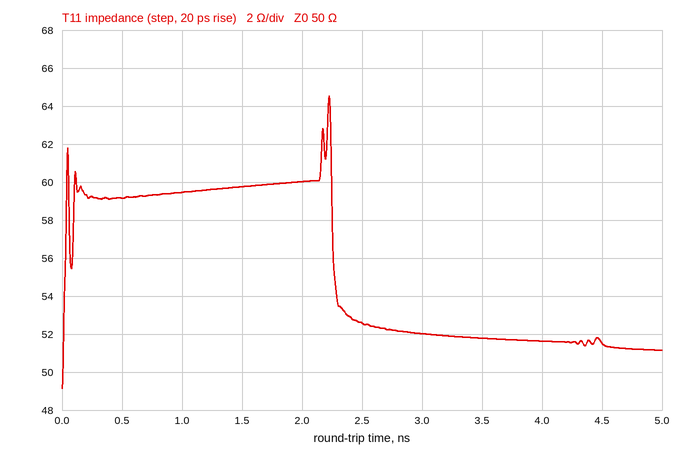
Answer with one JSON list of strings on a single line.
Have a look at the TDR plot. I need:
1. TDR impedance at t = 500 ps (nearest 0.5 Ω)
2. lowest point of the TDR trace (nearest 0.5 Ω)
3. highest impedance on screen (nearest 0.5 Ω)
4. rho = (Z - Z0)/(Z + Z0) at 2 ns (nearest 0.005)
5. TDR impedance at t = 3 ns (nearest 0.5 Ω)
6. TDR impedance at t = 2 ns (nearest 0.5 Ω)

["59.0 Ω", "49.0 Ω", "64.5 Ω", "+0.090", "52.0 Ω", "60.0 Ω"]
